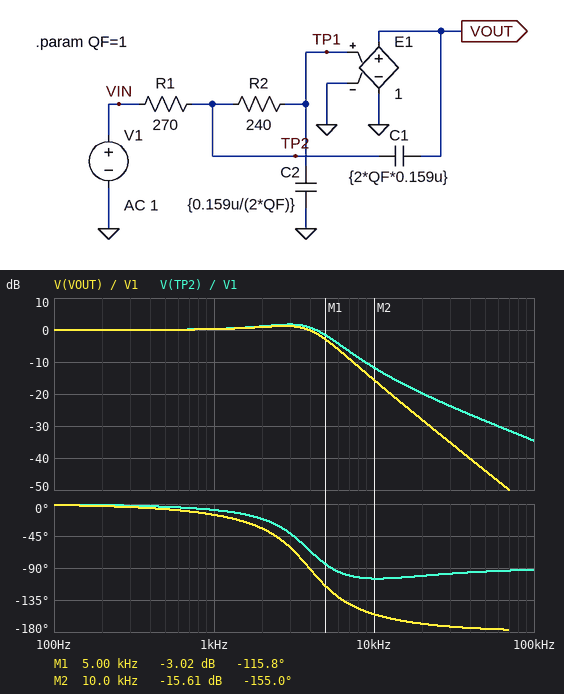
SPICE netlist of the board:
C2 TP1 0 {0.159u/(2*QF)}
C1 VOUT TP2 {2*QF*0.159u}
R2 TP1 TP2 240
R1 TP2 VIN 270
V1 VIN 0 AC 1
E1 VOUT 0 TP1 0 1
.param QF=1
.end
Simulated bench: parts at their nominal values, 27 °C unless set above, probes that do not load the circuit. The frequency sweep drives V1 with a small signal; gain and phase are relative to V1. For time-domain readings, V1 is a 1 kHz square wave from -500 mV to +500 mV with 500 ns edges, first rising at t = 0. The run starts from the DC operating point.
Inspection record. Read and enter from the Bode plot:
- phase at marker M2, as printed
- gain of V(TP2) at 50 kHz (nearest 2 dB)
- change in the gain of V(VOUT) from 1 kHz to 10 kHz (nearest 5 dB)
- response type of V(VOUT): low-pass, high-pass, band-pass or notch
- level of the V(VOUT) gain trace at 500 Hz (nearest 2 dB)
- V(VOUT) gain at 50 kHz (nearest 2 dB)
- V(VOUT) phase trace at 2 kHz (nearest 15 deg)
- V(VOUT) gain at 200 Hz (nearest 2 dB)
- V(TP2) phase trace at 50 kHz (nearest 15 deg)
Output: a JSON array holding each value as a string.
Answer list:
["-155.0 deg", "-28 dB", "-15 dB", "low-pass", "0 dB", "-44 dB", "-30 deg", "0 dB", "-90 deg"]
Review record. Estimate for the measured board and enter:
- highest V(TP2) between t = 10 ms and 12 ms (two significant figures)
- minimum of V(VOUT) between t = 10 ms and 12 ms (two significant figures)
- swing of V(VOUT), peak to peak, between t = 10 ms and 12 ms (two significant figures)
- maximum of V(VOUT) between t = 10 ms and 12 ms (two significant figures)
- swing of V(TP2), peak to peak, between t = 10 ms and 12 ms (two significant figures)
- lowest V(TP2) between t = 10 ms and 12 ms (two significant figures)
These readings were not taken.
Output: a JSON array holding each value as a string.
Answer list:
["690 mV", "-660 mV", "1.3 V", "660 mV", "1.4 V", "-690 mV"]
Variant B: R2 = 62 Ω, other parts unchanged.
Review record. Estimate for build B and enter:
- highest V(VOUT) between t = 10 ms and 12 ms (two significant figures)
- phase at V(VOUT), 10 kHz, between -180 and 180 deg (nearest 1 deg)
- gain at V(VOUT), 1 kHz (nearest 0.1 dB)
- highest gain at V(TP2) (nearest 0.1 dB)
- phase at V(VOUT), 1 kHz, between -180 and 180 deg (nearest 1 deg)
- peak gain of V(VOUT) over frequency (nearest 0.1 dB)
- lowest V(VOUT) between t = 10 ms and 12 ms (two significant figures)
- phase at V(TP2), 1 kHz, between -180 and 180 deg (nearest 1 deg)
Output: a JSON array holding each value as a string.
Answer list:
["570 mV", "-112 deg", "0 dB", "0.2 dB", "-10 deg", "0.1 dB", "-570 mV", "-8 deg"]
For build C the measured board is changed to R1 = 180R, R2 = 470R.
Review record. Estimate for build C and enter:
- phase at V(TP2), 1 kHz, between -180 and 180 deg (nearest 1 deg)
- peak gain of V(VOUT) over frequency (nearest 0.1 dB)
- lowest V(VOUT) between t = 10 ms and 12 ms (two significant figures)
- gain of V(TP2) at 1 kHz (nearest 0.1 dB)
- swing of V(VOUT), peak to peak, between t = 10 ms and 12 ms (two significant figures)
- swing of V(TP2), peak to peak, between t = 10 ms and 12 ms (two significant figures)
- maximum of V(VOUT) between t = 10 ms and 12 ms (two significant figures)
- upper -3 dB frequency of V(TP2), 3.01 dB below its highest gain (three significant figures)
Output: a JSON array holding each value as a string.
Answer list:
["-6 deg", "0.7 dB", "-620 mV", "0.5 dB", "1.2 V", "1.4 V", "620 mV", "4.59 kHz"]
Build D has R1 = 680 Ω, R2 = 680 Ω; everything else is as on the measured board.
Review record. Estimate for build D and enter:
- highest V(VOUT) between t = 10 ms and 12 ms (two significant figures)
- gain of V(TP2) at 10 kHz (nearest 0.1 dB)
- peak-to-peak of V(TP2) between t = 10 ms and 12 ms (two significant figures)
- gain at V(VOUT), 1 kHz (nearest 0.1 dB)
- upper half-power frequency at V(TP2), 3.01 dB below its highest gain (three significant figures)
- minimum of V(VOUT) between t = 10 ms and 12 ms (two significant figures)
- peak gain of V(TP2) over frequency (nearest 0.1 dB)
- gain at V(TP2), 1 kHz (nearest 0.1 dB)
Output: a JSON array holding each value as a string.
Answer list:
["680 mV", "-22.2 dB", "1.4 V", "1.2 dB", "1.83 kHz", "-680 mV", "1.8 dB", "1.7 dB"]
